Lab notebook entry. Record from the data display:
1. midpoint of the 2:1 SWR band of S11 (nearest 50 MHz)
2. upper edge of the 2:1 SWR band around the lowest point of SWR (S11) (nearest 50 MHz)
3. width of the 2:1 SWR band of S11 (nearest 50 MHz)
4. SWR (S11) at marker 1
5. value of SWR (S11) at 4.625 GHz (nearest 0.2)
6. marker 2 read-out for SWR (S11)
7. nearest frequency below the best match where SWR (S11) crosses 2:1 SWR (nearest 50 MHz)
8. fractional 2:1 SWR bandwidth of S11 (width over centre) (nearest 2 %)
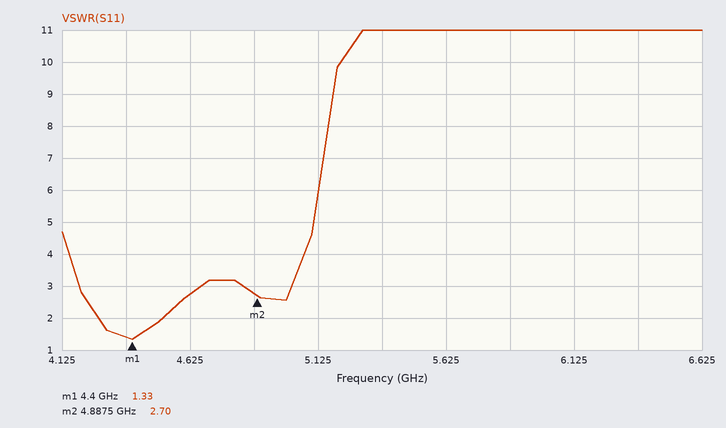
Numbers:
4.40 GHz
4.50 GHz
250 MHz
1.33
2.8
2.70
4.25 GHz
6 %
